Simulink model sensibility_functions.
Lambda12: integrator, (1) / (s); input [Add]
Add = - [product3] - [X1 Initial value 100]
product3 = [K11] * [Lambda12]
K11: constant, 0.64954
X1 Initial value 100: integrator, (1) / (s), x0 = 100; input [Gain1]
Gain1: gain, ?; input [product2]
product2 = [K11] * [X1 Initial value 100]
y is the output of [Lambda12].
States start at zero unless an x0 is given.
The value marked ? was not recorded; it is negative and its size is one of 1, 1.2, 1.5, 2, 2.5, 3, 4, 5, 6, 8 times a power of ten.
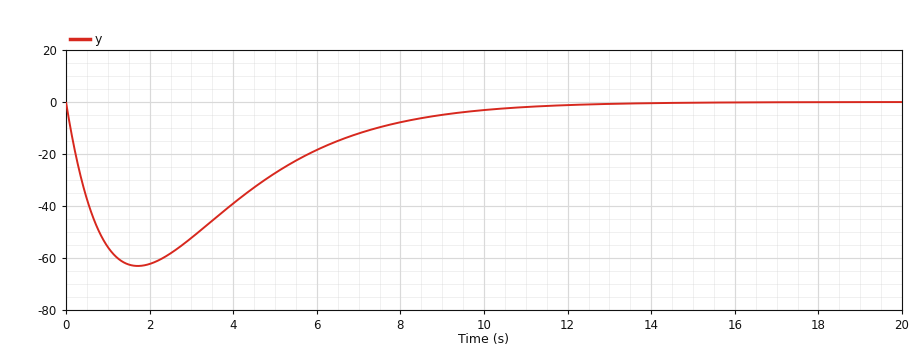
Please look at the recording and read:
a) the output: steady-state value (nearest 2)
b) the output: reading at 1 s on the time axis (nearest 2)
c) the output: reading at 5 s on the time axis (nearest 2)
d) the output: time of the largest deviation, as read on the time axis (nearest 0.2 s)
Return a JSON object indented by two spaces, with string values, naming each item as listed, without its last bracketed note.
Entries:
{
  "the output: steady-state value": "0",
  "the output: reading at 1 s on the time axis": "-56",
  "the output: reading at 5 s on the time axis": "-28",
  "the output: time of the largest deviation, as read on the time axis": "1.8 s"
}
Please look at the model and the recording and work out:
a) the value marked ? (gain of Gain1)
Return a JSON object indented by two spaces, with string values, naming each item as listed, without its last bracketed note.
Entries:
{
  "the value marked ?": "-0.8"
}
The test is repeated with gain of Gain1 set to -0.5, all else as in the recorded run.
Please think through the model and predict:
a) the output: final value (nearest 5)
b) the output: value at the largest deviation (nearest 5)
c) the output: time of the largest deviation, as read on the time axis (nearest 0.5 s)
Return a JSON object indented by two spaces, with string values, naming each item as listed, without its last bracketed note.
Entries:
{
  "the output: final value": "0",
  "the output: value at the largest deviation": "-75",
  "the output: time of the largest deviation, as read on the time axis": "2.0 s"
}
